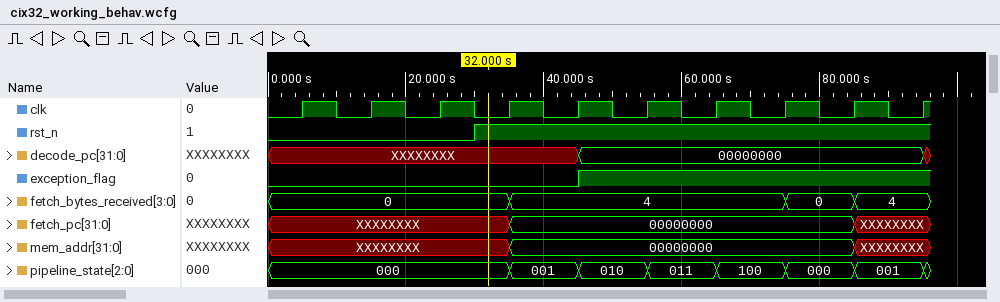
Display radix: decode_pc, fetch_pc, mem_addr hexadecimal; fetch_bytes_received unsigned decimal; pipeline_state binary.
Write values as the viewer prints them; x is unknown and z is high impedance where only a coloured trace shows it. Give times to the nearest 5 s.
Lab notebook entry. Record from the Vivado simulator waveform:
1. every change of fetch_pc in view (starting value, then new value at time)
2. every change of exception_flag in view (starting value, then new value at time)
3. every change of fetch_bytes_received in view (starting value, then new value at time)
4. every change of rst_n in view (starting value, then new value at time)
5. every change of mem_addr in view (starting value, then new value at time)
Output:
XXXXXXXX, 00000000 at 35 s, XXXXXXXX at 85 s
0, 1 at 45 s
0, 4 at 35 s, 0 at 75 s, 4 at 85 s
0, 1 at 30 s
XXXXXXXX, 00000000 at 35 s, XXXXXXXX at 85 s
